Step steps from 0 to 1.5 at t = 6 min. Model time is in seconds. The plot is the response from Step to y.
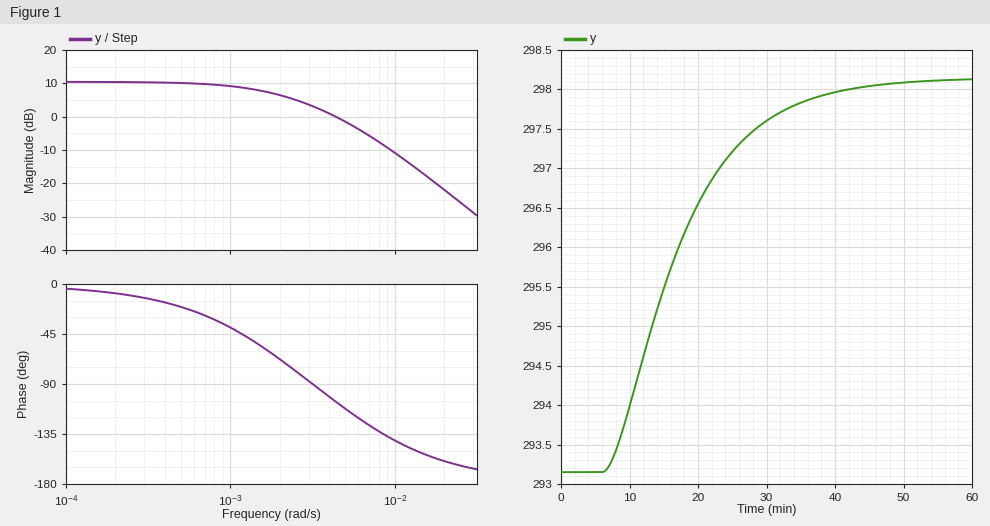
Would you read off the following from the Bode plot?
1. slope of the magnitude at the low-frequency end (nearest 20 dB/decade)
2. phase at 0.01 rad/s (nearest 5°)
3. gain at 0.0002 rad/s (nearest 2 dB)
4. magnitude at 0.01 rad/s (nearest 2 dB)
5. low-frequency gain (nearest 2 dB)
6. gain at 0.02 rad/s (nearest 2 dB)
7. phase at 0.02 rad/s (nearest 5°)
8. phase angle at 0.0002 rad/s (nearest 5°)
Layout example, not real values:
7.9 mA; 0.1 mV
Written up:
0 dB/decade; -140°; 10 dB; -10 dB; 10 dB; -22 dB; -160°; -10°
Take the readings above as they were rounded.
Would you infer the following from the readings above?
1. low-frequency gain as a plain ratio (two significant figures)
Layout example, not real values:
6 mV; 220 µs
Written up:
3.2
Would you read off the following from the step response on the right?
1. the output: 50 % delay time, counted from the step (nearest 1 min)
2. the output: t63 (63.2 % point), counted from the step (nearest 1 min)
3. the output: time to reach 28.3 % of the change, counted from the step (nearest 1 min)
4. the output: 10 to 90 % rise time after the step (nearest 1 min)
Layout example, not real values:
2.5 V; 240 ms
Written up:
10 min; 13 min; 6 min; 22 min
